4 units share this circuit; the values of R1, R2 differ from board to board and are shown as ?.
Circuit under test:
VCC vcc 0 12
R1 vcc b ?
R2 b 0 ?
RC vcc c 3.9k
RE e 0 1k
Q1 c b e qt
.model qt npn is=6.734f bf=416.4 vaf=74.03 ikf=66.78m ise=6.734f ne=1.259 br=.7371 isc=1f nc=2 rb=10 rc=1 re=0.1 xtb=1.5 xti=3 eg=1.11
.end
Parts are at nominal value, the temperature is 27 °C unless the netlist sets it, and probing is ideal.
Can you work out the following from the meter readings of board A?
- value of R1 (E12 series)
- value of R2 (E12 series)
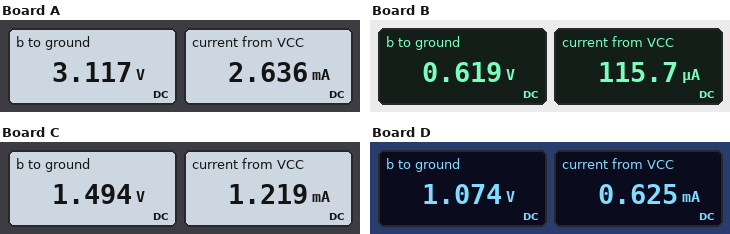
39 kΩ
15 kΩ
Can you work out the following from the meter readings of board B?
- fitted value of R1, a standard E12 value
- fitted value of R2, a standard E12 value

150 kΩ
8.2 kΩ
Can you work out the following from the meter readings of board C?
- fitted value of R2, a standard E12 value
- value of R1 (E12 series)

3.9 kΩ
27 kΩ
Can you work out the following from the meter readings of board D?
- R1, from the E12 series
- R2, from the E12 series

56 kΩ
5.6 kΩ
